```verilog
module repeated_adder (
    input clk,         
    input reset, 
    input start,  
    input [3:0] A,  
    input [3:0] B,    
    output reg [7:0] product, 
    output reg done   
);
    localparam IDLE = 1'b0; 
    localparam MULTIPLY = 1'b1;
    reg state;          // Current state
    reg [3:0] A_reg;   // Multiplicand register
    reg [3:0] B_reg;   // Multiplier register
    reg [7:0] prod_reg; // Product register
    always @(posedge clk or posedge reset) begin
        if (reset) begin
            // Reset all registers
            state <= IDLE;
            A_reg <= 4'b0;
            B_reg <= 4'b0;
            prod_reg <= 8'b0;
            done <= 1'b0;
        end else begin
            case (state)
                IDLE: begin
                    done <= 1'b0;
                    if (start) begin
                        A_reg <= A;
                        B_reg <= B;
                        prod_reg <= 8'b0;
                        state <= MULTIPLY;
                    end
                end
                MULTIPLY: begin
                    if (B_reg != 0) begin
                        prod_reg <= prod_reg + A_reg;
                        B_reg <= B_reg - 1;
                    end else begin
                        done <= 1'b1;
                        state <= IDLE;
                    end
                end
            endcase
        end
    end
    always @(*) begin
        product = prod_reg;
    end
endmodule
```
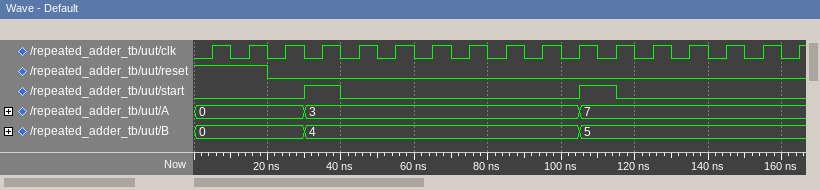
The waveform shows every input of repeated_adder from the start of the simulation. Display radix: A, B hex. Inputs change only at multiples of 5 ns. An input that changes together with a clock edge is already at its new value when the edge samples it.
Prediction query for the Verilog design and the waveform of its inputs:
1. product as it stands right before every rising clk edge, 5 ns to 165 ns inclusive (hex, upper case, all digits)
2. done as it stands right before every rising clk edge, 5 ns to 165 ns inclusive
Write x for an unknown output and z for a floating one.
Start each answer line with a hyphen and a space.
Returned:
- 00, 00, 00, 00, 00, 03, 06, 09, 0C, 0C, 0C, 00, 07, 0E, 15, 1C, 23
- 0 0 0 0 0 0 0 0 0 1 0 0 0 0 0 0 0
